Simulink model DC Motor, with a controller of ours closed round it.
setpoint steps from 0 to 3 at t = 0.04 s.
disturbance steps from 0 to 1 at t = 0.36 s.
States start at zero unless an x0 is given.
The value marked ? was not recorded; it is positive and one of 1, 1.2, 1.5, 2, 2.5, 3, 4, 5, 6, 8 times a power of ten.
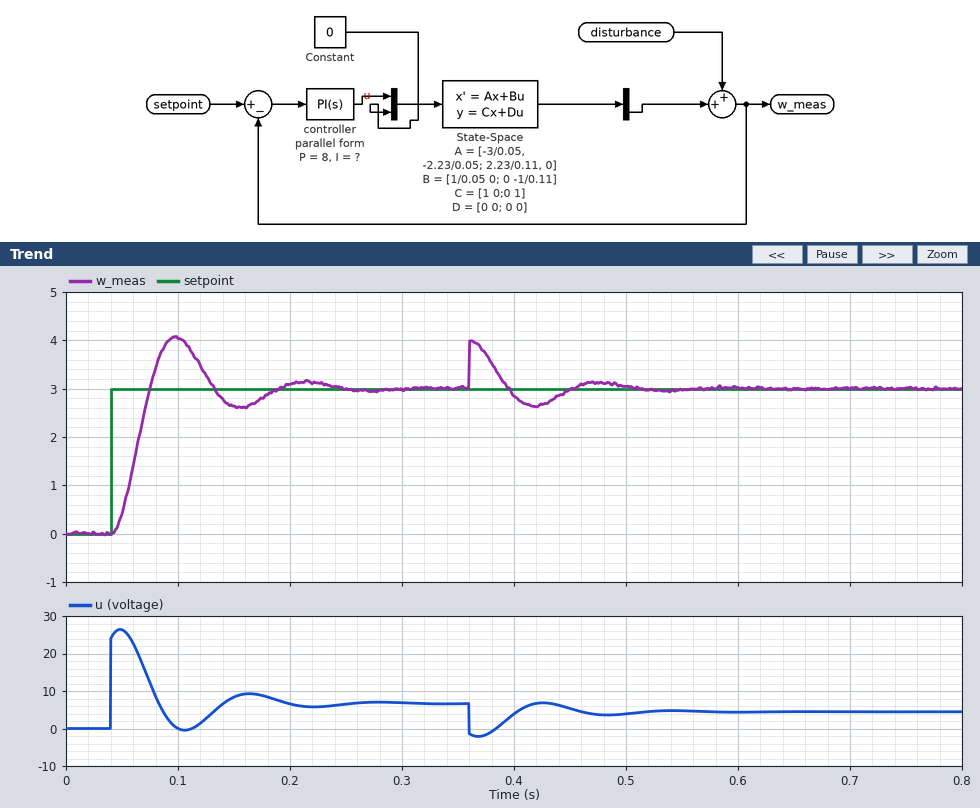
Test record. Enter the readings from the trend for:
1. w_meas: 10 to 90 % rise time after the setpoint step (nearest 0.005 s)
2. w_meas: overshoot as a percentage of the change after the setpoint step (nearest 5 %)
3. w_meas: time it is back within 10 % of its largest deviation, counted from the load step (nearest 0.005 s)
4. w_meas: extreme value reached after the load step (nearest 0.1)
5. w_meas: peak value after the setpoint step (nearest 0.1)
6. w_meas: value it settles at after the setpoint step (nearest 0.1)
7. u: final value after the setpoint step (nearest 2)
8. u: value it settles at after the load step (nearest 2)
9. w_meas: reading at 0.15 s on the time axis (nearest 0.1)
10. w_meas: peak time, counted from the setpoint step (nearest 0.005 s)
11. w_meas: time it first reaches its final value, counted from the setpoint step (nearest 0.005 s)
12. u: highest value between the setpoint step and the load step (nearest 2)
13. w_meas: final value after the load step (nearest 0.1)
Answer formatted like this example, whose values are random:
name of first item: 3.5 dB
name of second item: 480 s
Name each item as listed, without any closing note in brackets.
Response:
w_meas: 10 to 90 % rise time after the setpoint step: 0.025 s
w_meas: overshoot as a percentage of the change after the setpoint step: 35 %
w_meas: time it is back within 10 % of its largest deviation, counted from the load step: 0.130 s
w_meas: extreme value reached after the load step: 4.0
w_meas: peak value after the setpoint step: 4.1
w_meas: value it settles at after the setpoint step: 3.0
u: final value after the setpoint step: 6
u: value it settles at after the load step: 4
w_meas: reading at 0.15 s on the time axis: 2.6
w_meas: peak time, counted from the setpoint step: 0.060 s
w_meas: time it first reaches its final value, counted from the setpoint step: 0.035 s
u: highest value between the setpoint step and the load step: 26
w_meas: final value after the load step: 3.0
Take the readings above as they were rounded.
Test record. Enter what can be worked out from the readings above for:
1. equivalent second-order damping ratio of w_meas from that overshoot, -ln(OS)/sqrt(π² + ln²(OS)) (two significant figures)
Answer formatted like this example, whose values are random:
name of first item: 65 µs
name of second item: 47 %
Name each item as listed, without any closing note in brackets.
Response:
equivalent second-order damping ratio of w_meas from that overshoot, -ln(OS)/sqrt(π² + ln²(OS)): 0.32
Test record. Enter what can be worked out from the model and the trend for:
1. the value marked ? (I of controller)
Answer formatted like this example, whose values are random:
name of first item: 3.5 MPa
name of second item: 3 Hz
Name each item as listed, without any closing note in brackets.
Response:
the value marked ?: 200
